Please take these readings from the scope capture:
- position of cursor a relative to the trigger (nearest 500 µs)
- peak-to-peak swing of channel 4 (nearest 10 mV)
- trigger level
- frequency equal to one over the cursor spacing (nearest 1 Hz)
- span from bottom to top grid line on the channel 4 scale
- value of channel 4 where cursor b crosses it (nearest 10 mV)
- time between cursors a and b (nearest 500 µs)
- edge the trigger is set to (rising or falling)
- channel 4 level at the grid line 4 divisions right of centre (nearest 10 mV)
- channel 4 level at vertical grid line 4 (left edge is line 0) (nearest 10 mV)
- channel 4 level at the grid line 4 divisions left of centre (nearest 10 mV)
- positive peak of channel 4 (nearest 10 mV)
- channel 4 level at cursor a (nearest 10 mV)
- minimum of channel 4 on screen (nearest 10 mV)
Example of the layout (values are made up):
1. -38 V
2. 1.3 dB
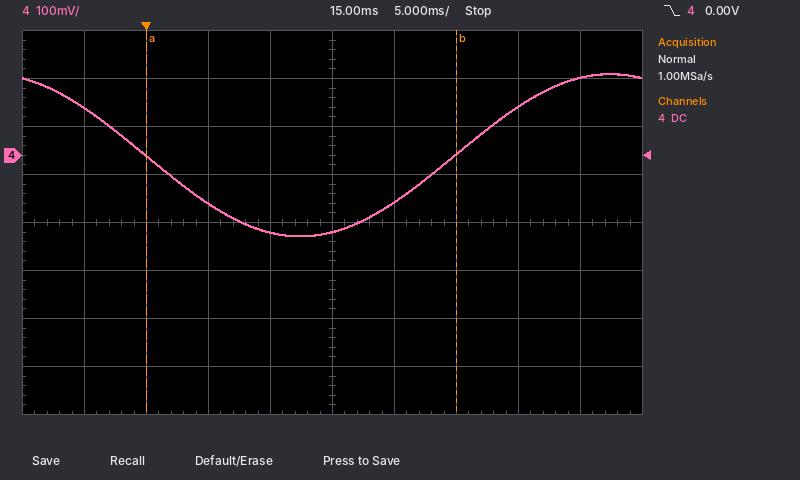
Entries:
1. 0.0 ms
2. 340 mV
3. 0.00 V
4. 40 Hz
5. 800 mV
6. 0 mV
7. 25.0 ms
8. falling
9. 160 mV
10. -160 mV
11. 100 mV
12. 170 mV
13. 0 mV
14. -170 mV
